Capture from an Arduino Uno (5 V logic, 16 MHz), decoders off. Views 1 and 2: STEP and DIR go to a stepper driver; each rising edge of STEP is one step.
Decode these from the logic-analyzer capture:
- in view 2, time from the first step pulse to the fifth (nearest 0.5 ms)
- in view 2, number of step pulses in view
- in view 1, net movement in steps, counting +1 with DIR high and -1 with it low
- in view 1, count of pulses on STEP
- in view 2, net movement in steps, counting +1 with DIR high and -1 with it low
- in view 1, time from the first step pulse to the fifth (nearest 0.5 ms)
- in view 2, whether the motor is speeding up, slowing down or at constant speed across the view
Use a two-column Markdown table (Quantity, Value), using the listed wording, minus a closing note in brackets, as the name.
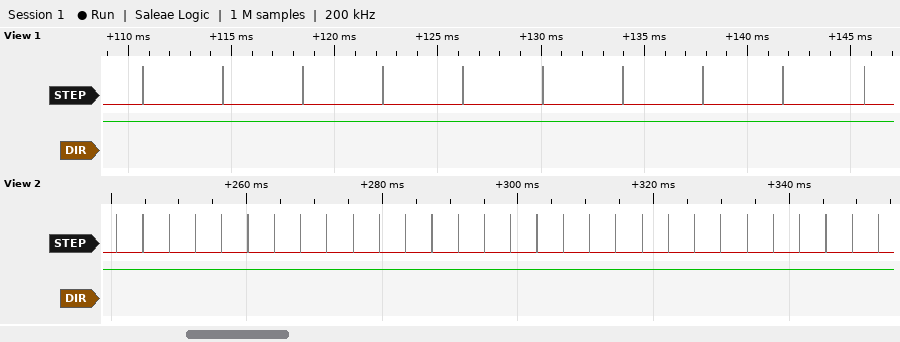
| Quantity | Value |
|---|---|
| in view 2, time from the first step pulse to the fifth | 15.5 ms |
| in view 2, number of step pulses in view | 30 |
| in view 1, net movement in steps, counting +1 with DIR high and -1 with it low | +10 |
| in view 1, count of pulses on STEP | 10 |
| in view 2, net movement in steps, counting +1 with DIR high and -1 with it low | +30 |
| in view 1, time from the first step pulse to the fifth | 15.5 ms |
| in view 2, whether the motor is speeding up, slowing down or at constant speed across the view | constant speed |
